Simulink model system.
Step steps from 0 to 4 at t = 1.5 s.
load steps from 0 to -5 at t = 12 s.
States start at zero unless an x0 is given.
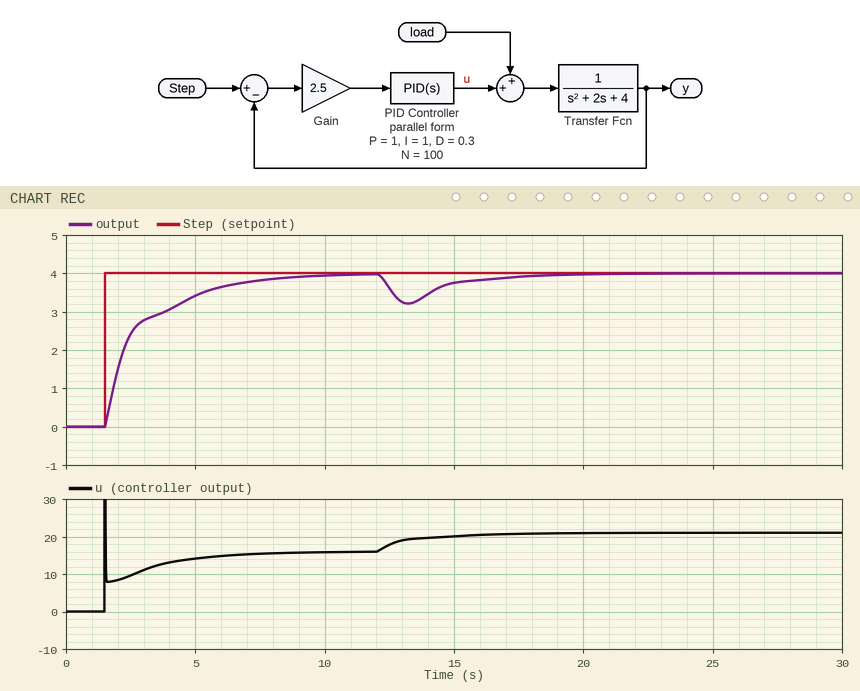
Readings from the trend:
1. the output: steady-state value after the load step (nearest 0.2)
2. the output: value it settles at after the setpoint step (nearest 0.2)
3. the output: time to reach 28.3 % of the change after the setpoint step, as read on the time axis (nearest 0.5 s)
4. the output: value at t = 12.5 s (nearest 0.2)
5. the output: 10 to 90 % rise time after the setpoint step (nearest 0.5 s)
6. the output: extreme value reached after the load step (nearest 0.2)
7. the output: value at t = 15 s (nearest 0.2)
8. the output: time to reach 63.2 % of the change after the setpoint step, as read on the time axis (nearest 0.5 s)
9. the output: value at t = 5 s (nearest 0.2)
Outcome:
4.0
4.0
2.0 s
3.6
4.0 s
3.2
3.8
2.5 s
3.4
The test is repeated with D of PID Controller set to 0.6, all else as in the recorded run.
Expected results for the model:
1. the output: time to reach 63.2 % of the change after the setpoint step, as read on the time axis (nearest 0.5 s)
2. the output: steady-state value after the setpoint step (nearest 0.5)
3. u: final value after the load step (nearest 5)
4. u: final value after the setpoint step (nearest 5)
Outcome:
3.0 s
4.0
20
15
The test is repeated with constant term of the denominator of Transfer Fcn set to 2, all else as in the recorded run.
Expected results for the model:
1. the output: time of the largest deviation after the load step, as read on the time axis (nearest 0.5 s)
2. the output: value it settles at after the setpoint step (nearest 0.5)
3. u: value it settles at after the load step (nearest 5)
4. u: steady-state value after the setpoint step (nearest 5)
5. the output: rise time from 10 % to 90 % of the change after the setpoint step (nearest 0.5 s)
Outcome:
13.5 s
4.0
15
10
1.5 s
